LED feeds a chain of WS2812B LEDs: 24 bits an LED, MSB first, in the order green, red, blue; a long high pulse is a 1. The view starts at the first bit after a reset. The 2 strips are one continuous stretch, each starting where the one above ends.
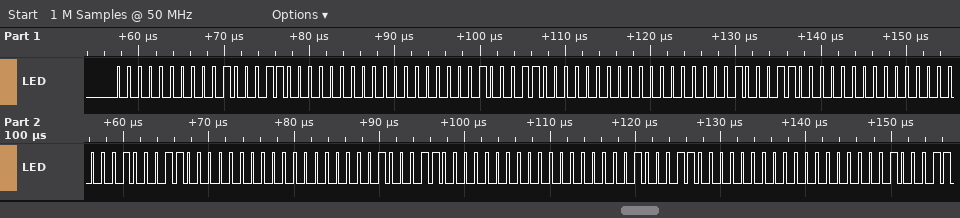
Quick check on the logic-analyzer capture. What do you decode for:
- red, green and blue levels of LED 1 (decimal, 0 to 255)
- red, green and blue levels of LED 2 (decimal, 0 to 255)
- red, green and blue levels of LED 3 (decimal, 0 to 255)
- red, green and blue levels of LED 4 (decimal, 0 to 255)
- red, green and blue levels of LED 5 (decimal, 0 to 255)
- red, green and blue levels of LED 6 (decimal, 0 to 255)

35, 0, 0
35, 0, 0
35, 0, 0
35, 0, 0
35, 0, 0
35, 0, 0
